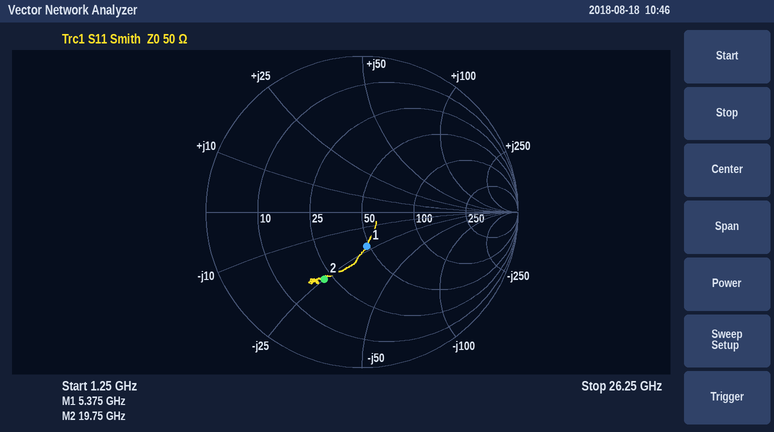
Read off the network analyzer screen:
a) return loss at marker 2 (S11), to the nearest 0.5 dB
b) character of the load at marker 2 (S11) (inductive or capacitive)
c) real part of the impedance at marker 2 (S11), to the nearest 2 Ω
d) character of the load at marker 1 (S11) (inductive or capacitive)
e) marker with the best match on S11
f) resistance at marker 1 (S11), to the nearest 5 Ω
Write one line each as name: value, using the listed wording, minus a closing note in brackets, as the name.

return loss at marker 2 (S11), to the nearest 0.5 dB: 6.0 dB
character of the load at marker 2 (S11): capacitive
real part of the impedance at marker 2 (S11), to the nearest 2 Ω: 22 Ω
character of the load at marker 1 (S11): capacitive
marker with the best match on S11: marker 1
resistance at marker 1 (S11), to the nearest 5 Ω: 50 Ω
